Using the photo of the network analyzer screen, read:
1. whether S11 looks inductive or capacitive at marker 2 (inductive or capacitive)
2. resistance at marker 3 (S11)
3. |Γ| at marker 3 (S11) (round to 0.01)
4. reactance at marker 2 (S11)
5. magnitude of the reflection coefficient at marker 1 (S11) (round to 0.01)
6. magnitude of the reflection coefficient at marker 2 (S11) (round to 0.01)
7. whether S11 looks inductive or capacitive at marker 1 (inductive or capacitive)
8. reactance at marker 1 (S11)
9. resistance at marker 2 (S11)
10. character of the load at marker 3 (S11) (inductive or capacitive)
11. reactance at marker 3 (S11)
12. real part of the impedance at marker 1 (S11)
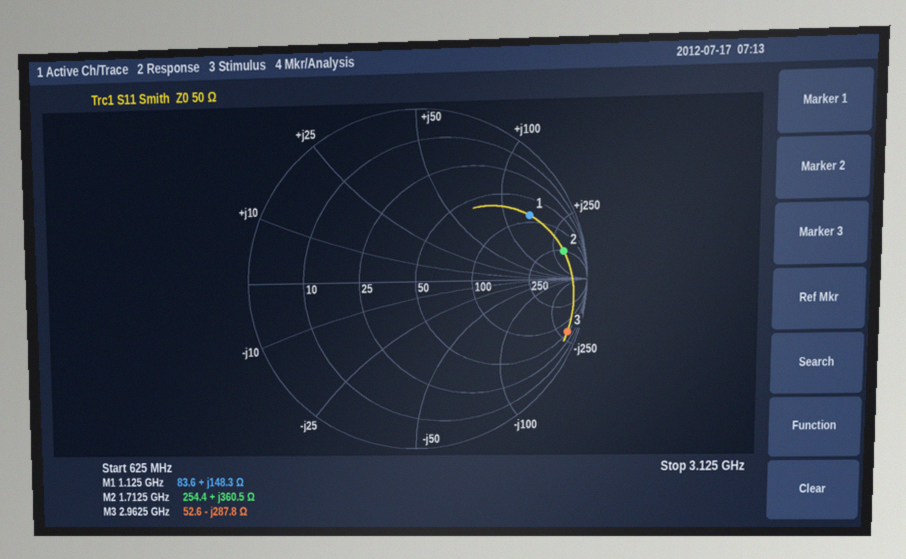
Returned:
inductive
52.6 Ω
0.94
+360.5 Ω
0.76
0.88
inductive
+148.3 Ω
254.4 Ω
capacitive
-287.8 Ω
83.6 Ω
